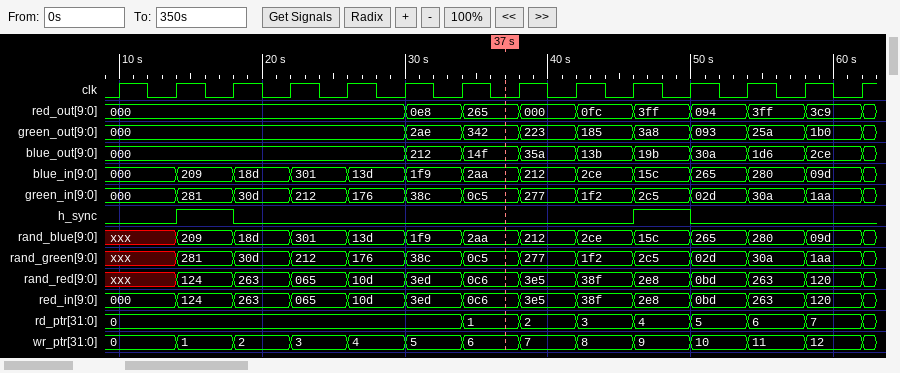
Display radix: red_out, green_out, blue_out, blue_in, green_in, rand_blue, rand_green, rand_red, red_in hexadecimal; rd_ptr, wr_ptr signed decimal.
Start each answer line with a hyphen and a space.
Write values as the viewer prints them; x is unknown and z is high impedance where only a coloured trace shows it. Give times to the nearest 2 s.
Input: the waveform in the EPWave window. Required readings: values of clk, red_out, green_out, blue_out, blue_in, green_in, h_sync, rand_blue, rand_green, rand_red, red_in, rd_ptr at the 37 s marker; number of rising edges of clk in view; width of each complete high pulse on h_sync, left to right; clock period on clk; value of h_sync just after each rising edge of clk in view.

- clk=0, red_out=265, green_out=342, blue_out=14f, blue_in=2aa, green_in=0c5, h_sync=0, rand_blue=2aa, rand_green=0c5, rand_red=0c6, red_in=0c6, rd_ptr=1
- 14
- 4 s, 4 s
- 4 s
- 0 1 0 0 0 0 0 0 0 1 0 0 0 0
